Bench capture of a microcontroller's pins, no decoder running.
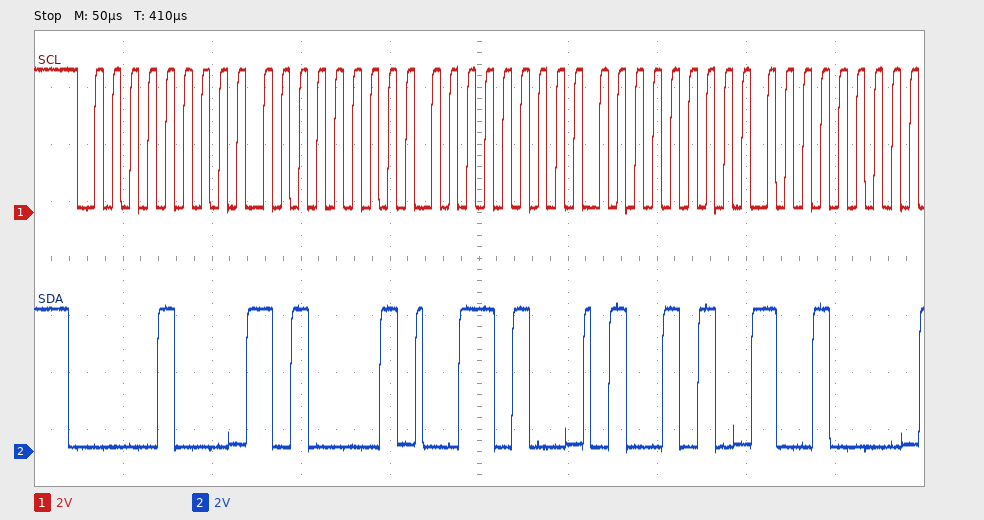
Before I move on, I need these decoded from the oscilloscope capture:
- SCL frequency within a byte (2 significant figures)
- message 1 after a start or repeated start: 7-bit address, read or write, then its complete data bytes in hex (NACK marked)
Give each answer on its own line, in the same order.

100 kHz
0x04 write: A1 34 4A 90
